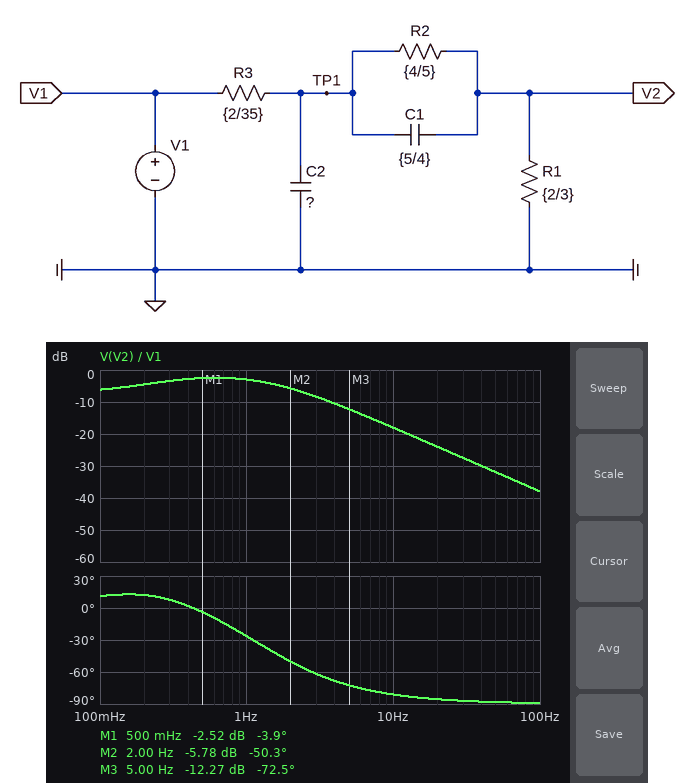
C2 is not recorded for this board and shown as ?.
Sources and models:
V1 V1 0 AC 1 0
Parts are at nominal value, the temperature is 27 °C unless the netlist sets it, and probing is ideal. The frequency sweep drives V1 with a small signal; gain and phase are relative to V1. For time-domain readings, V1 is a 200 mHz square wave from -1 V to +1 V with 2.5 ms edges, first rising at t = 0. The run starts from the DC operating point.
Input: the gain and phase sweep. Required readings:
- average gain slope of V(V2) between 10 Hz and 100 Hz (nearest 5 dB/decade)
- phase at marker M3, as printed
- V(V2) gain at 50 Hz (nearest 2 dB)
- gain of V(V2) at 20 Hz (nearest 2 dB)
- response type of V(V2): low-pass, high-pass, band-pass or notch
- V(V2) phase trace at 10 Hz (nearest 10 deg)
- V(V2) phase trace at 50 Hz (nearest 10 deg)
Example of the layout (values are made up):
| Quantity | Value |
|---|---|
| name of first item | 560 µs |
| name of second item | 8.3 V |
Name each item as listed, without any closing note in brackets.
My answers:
| Quantity | Value |
|---|---|
| average gain slope of V(V2) between 10 Hz and 100 Hz | -20 dB/decade |
| phase at marker M3, as printed | -72.5 deg |
| V(V2) gain at 50 Hz | -32 dB |
| gain of V(V2) at 20 Hz | -24 dB |
| response type of V(V2): low-pass, high-pass, band-pass or notch | low-pass |
| V(V2) phase trace at 10 Hz | -80 deg |
| V(V2) phase trace at 50 Hz | -90 deg |
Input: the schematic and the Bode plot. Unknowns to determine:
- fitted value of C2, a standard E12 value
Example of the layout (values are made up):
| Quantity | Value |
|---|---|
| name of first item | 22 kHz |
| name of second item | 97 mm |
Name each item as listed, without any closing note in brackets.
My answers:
| Quantity | Value |
|---|---|
| fitted value of C2, a standard E12 value | 2.2 F |
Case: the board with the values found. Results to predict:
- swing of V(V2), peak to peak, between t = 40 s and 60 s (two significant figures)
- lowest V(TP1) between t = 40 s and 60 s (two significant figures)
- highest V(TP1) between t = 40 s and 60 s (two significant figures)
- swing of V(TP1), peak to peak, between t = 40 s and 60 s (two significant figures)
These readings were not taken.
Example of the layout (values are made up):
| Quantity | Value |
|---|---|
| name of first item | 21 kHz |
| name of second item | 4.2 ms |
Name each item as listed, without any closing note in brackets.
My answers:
| Quantity | Value |
|---|---|
| swing of V(V2), peak to peak, between t = 40 s and 60 s | 1.9 V |
| lowest V(TP1) between t = 40 s and 60 s | -960 mV |
| highest V(TP1) between t = 40 s and 60 s | 960 mV |
| swing of V(TP1), peak to peak, between t = 40 s and 60 s | 1.9 V |
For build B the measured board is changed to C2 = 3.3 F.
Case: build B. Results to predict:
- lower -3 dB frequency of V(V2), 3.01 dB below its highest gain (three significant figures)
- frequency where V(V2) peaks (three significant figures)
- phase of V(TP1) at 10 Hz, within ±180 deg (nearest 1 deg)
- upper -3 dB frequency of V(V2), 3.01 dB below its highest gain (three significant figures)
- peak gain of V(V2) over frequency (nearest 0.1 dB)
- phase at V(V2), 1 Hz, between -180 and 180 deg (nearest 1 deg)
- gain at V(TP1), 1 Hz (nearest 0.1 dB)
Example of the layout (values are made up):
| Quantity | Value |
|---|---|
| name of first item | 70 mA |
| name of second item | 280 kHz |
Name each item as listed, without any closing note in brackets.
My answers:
| Quantity | Value |
|---|---|
| lower -3 dB frequency of V(V2), 3.01 dB below its highest gain | 101 mHz |
| frequency where V(V2) peaks | 489 mHz |
| phase of V(TP1) at 10 Hz, within ±180 deg | -85 deg |
| upper -3 dB frequency of V(V2), 3.01 dB below its highest gain | 1.39 Hz |
| peak gain of V(V2) over frequency | -3.1 dB |
| phase at V(V2), 1 Hz, between -180 and 180 deg | -38 deg |
| gain at V(TP1), 1 Hz | -4.2 dB |
